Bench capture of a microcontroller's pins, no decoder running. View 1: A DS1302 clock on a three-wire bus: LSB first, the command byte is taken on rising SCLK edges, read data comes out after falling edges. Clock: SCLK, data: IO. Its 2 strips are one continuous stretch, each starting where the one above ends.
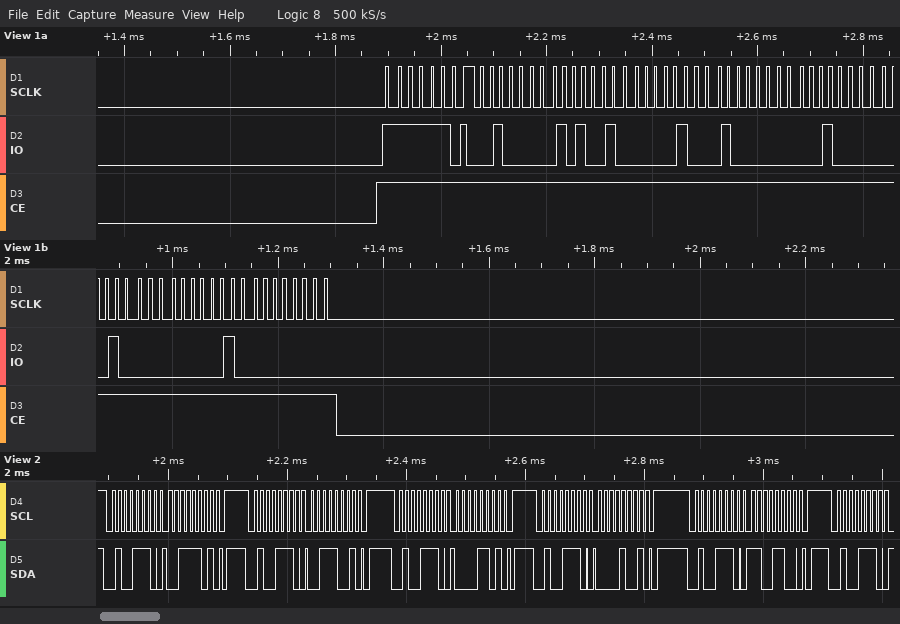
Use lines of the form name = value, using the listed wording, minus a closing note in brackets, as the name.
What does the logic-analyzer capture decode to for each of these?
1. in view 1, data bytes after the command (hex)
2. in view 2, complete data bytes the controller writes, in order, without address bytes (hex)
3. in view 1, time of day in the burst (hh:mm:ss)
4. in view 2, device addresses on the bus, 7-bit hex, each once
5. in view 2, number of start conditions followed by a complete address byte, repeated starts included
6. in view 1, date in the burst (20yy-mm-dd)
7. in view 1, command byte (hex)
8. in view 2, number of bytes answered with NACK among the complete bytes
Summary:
in view 1, data bytes after the command = 04 25 10 01 04 04 20 00
in view 2, complete data bytes the controller writes, in order, without address bytes = 3D 39 0D 09 CC
in view 1, time of day in the burst = 10:25:04
in view 2, device addresses on the bus, 7-bit hex, each once = 0x27
in view 2, number of start conditions followed by a complete address byte, repeated starts included = 6
in view 1, date in the burst = 2020-04-01
in view 1, command byte = 0xBF
in view 2, number of bytes answered with NACK among the complete bytes = 0
